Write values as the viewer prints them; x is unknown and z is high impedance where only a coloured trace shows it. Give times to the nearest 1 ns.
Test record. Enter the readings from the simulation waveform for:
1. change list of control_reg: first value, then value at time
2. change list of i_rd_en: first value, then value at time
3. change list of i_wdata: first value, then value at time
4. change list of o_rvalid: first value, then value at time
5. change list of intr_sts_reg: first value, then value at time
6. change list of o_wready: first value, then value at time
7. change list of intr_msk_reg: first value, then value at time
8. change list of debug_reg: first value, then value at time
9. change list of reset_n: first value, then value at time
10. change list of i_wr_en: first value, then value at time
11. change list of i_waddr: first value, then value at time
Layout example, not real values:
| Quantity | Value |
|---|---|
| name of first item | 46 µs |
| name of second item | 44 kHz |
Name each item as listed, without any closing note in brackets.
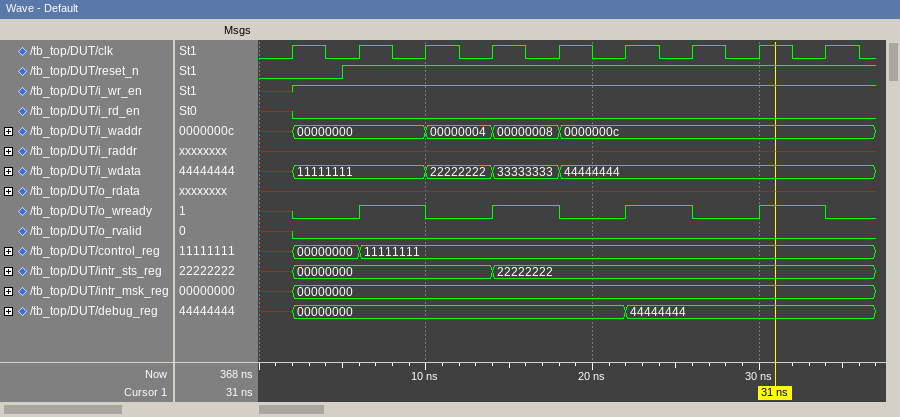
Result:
| Quantity | Value |
|---|---|
| change list of control_reg: first value, then value at time | x, 00000000 at 2 ns, 11111111 at 6 ns |
| change list of i_rd_en: first value, then value at time | x, 0 at 2 ns |
| change list of i_wdata: first value, then value at time | x, 11111111 at 2 ns, 22222222 at 10 ns, 33333333 at 14 ns, 44444444 at 18 ns |
| change list of o_rvalid: first value, then value at time | x, 0 at 2 ns |
| change list of intr_sts_reg: first value, then value at time | x, 00000000 at 2 ns, 22222222 at 14 ns |
| change list of o_wready: first value, then value at time | x, 0 at 2 ns, 1 at 6 ns, 0 at 10 ns, 1 at 14 ns, 0 at 18 ns, 1 at 22 ns, 0 at 26 ns, 1 at 30 ns, 0 at 34 ns |
| change list of intr_msk_reg: first value, then value at time | x, 00000000 at 2 ns |
| change list of debug_reg: first value, then value at time | x, 00000000 at 2 ns, 44444444 at 22 ns |
| change list of reset_n: first value, then value at time | 0, 1 at 5 ns |
| change list of i_wr_en: first value, then value at time | x, 1 at 2 ns |
| change list of i_waddr: first value, then value at time | x, 00000000 at 2 ns, 00000004 at 10 ns, 00000008 at 14 ns, 0000000c at 18 ns |
